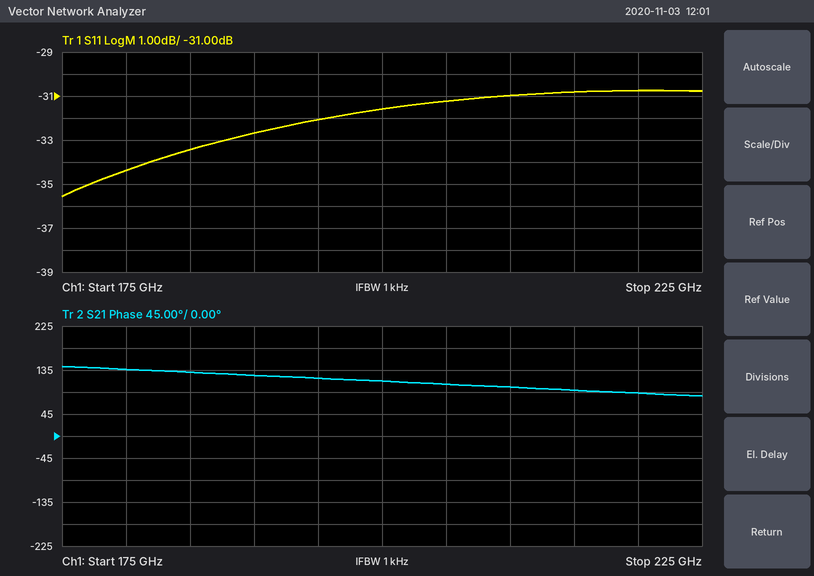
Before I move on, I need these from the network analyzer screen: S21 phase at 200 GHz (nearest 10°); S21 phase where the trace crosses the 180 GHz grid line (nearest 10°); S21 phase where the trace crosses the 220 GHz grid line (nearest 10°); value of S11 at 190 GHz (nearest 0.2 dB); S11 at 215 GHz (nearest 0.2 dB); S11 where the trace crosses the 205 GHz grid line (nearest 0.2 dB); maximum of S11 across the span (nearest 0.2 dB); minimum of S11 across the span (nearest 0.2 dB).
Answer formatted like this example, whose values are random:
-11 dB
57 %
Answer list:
110°
140°
90°
-32.6 dB
-30.8 dB
-31.2 dB
-30.8 dB
-35.6 dB
